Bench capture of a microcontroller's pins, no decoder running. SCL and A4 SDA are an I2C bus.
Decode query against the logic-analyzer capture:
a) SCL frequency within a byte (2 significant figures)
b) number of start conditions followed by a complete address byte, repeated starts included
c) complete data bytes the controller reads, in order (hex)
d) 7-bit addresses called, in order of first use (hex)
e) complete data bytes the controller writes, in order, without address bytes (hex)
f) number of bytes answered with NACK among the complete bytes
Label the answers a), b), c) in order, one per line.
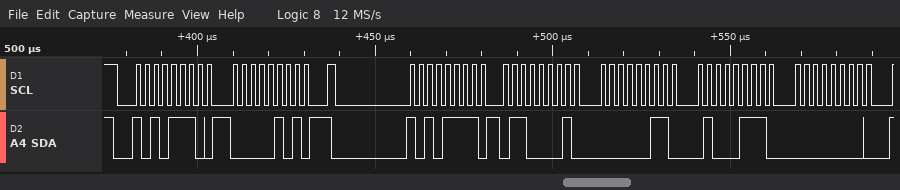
a) 400 kHz
b) 2
c) 61 03 47 00
d) 0x57
e) 05
f) 0
